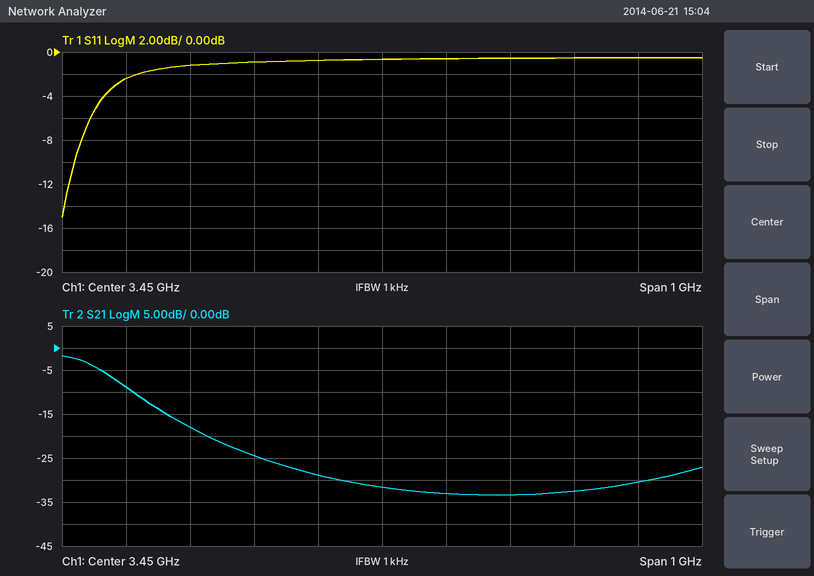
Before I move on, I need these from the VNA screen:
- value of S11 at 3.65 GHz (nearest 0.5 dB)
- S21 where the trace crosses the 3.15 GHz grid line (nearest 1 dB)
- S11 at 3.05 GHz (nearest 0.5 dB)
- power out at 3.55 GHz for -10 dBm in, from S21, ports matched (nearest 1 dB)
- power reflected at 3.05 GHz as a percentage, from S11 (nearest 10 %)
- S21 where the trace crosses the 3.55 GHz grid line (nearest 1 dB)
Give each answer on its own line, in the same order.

-0.5 dB
-18 dB
-2.5 dB
-43 dBm
60 %
-33 dB
